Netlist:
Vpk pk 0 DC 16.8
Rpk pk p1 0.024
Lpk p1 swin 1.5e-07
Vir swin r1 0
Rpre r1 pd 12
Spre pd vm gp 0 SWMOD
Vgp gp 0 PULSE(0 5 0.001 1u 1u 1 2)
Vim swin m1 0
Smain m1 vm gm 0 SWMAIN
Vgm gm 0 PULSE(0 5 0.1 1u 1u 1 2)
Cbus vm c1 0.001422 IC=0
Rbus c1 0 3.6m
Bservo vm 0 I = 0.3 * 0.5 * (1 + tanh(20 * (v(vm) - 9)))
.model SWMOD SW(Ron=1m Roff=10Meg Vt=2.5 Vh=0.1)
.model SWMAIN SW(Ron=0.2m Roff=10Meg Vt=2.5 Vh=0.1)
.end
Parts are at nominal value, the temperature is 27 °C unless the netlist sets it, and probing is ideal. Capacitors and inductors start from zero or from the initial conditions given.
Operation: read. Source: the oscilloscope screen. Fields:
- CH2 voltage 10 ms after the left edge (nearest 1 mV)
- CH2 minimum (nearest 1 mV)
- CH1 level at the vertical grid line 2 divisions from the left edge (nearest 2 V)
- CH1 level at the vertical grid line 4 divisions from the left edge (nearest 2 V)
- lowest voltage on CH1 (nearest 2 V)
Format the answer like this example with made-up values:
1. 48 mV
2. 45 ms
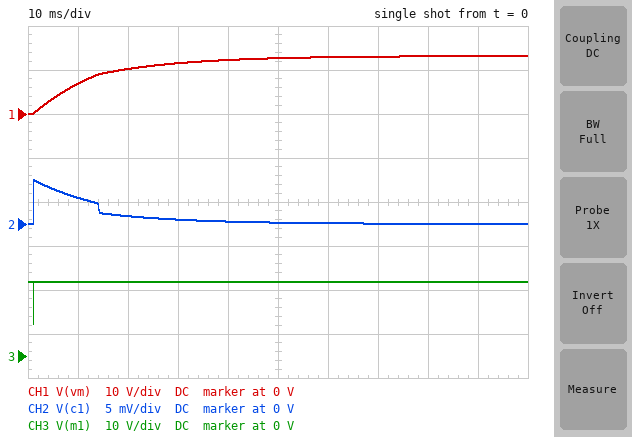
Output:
1. 3 mV
2. 0 V
3. 10 V
4. 12 V
5. 0 V
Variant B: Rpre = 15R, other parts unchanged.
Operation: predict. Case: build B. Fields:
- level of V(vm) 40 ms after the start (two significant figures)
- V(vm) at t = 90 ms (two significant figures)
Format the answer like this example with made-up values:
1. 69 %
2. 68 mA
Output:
1. 11 V
2. 12 V
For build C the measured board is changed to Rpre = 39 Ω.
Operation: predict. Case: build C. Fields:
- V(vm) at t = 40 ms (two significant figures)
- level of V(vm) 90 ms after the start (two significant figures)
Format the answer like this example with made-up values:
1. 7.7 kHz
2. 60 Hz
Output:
1. 8.5 V
2. 9.0 V
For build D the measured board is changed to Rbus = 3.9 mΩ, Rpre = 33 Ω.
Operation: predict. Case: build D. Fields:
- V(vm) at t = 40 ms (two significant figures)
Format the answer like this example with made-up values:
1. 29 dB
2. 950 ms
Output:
1. 9.0 V
